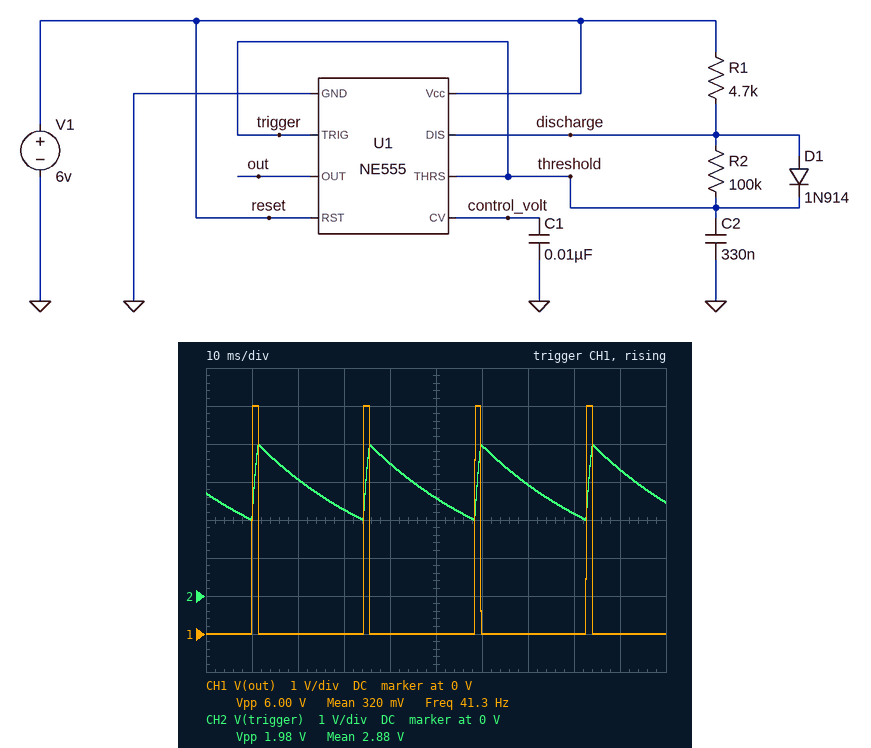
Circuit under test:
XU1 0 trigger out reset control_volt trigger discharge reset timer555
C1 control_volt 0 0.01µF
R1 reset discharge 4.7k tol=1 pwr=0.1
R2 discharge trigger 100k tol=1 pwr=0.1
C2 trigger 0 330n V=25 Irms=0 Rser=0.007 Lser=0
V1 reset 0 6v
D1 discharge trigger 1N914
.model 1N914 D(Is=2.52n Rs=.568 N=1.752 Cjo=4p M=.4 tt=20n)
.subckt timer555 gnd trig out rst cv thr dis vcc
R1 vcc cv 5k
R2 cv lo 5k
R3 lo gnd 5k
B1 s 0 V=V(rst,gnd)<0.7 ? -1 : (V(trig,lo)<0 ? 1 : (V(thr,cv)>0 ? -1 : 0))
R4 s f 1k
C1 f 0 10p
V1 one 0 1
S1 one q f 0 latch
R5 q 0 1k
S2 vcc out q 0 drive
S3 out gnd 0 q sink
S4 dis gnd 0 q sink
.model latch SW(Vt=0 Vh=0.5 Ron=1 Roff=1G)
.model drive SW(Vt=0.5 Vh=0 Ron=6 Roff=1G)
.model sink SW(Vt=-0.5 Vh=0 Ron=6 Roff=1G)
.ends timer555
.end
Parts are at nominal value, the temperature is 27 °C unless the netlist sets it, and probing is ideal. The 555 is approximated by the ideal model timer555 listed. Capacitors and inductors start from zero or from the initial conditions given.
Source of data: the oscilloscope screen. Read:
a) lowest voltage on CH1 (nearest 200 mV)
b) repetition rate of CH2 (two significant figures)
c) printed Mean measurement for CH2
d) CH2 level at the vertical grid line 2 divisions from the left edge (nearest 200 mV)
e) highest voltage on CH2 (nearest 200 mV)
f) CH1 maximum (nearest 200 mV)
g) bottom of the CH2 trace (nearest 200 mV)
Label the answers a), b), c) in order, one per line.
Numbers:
a) 0 V
b) 41 Hz
c) 2.88 V
d) 3.0 V
e) 4.0 V
f) 6.0 V
g) 2.0 V
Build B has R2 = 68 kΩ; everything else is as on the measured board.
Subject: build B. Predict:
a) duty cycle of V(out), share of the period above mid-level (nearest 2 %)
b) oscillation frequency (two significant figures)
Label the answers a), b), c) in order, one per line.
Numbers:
a) 8 %
b) 59 Hz
